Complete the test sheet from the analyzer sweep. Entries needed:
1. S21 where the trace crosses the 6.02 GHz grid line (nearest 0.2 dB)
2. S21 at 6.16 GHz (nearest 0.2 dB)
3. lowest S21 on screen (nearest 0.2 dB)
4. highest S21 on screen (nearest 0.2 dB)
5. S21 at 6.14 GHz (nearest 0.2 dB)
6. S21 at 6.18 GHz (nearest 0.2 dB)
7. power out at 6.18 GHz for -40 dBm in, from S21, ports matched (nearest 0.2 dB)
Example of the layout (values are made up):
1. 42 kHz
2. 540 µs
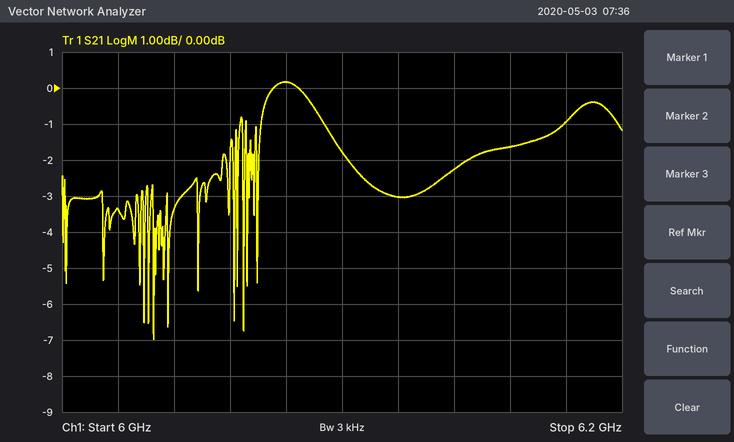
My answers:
1. -3.4 dB
2. -1.6 dB
3. -7.0 dB
4. 0.2 dB
5. -2.2 dB
6. -1.0 dB
7. -41.0 dBm
